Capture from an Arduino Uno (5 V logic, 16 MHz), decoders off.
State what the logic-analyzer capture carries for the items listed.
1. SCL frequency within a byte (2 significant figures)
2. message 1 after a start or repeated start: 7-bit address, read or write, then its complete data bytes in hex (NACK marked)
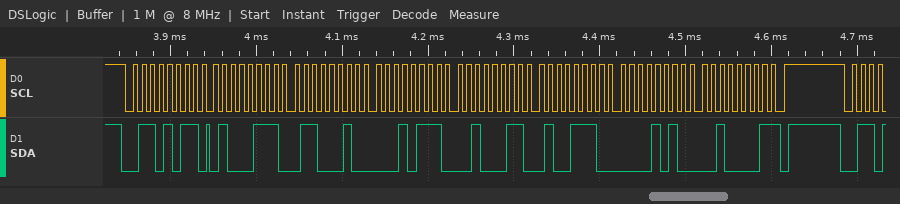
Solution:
100 kHz
0x35 read: 47 62 17 23 4E 0A 21 NACK
